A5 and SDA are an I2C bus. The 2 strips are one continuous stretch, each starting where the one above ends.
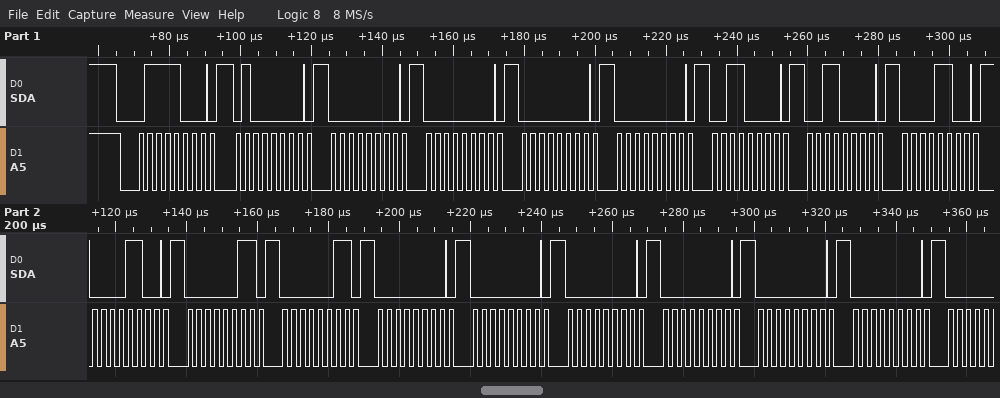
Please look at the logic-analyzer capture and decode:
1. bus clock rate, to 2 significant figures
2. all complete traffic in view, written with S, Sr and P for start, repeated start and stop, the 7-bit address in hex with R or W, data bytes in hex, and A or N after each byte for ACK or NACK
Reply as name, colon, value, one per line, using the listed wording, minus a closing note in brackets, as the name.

bus clock rate, to 2 significant figures: 400 kHz
all complete traffic in view, written with S, Sr and P for start, repeated start and stop, the 7-bit address in hex with R or W, data bytes in hex, and A or N after each byte for ACK or NACK: S 3CW A 40 A 00 A 00 A 00 A 00 A 30 A 30 A 0C A 0C A 03 A 03 A 00 A 00 A 00 A 00 A 00 A 00 A
